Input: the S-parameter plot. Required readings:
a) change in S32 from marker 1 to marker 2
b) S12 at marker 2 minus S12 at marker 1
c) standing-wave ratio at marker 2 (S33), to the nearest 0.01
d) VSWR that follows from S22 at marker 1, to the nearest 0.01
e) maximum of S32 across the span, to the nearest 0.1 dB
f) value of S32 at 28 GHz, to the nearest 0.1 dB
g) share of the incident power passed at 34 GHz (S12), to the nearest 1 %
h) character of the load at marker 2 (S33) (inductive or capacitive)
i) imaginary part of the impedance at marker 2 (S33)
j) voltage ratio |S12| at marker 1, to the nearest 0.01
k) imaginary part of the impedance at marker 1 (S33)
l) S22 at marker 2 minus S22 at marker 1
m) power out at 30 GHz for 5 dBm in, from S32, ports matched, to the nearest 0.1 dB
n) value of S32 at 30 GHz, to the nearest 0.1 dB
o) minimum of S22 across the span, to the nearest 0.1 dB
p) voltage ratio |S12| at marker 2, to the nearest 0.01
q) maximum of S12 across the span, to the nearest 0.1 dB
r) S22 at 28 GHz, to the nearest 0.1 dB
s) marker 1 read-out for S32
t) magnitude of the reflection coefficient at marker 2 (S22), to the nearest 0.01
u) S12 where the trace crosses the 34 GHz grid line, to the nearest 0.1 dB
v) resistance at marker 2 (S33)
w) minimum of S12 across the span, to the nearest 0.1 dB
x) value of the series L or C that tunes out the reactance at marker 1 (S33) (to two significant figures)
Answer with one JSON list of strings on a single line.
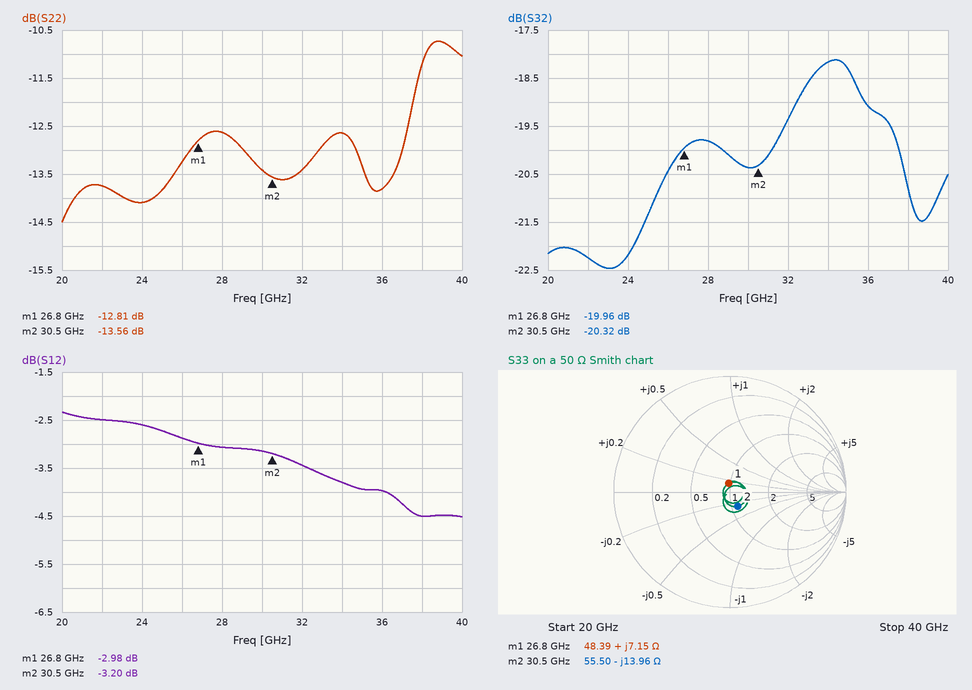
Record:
["-0.36 dB", "-0.22 dB", "1.33", "1.59", "-18.1 dB", "-19.8 dB", "42 %", "capacitive", "-13.96 Ω", "0.71", "+7.15 Ω", "-0.75 dB", "-15.4 dBm", "-20.4 dB", "-14.5 dB", "0.69", "-2.3 dB", "-12.6 dB", "-19.96 dB", "0.21", "-3.8 dB", "55.50 Ω", "-4.5 dB", "830 fF"]
